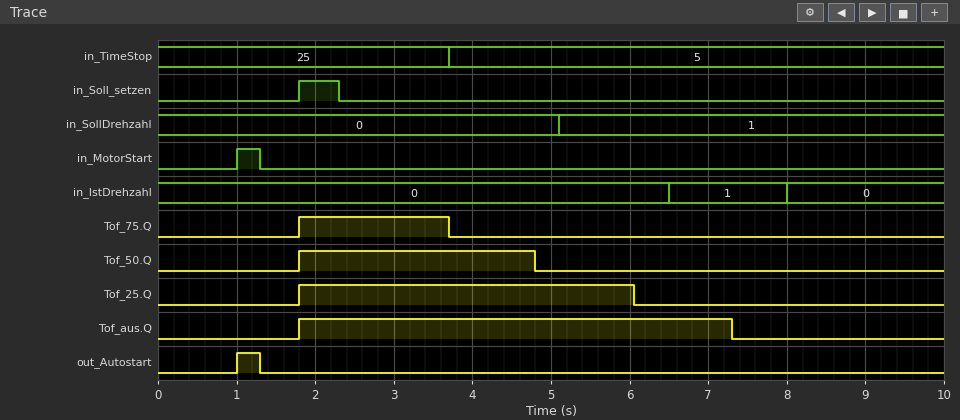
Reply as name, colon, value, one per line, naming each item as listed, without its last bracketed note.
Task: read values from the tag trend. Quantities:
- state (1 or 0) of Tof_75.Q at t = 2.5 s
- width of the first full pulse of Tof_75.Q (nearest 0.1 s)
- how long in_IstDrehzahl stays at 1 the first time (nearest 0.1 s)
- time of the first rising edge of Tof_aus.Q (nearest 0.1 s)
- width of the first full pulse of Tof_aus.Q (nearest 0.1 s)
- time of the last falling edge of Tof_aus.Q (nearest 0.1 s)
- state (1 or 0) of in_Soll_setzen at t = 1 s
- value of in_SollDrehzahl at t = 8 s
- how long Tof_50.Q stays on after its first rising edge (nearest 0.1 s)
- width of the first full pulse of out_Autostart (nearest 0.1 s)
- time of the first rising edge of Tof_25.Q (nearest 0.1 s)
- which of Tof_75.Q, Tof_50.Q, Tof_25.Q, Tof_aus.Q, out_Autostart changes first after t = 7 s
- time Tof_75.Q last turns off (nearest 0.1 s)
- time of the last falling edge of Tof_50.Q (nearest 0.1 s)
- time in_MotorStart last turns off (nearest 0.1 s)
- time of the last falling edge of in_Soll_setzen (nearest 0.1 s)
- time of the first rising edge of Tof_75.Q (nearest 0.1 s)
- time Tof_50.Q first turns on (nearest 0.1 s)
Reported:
state (1 or 0) of Tof_75.Q at t = 2.5 s: 1
width of the first full pulse of Tof_75.Q: 1.9 s
how long in_IstDrehzahl stays at 1 the first time: 1.5 s
time of the first rising edge of Tof_aus.Q: 1.8 s
width of the first full pulse of Tof_aus.Q: 5.5 s
time of the last falling edge of Tof_aus.Q: 7.3 s
state (1 or 0) of in_Soll_setzen at t = 1 s: 0
value of in_SollDrehzahl at t = 8 s: 1
how long Tof_50.Q stays on after its first rising edge: 3.0 s
width of the first full pulse of out_Autostart: 0.3 s
time of the first rising edge of Tof_25.Q: 1.8 s
which of Tof_75.Q, Tof_50.Q, Tof_25.Q, Tof_aus.Q, out_Autostart changes first after t = 7 s: Tof_aus.Q
time Tof_75.Q last turns off: 3.7 s
time of the last falling edge of Tof_50.Q: 4.8 s
time in_MotorStart last turns off: 1.3 s
time of the last falling edge of in_Soll_setzen: 2.3 s
time of the first rising edge of Tof_75.Q: 1.8 s
time Tof_50.Q first turns on: 1.8 s
